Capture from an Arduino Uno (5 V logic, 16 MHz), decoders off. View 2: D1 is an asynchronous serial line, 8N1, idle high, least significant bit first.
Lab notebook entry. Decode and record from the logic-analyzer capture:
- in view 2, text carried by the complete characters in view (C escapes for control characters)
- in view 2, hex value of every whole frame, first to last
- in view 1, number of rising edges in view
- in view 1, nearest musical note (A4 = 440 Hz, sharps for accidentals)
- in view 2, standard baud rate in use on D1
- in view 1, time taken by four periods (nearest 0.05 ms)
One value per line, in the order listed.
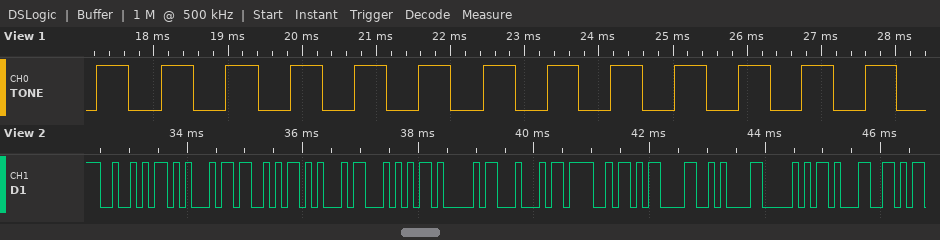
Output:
"RESETADO\r\nP1"
0x52 0x45 0x53 0x45 0x54 0x41 0x44 0x4F 0x0D 0x0A 0x50 0x31
13
D6
9600 baud
3.45 ms
